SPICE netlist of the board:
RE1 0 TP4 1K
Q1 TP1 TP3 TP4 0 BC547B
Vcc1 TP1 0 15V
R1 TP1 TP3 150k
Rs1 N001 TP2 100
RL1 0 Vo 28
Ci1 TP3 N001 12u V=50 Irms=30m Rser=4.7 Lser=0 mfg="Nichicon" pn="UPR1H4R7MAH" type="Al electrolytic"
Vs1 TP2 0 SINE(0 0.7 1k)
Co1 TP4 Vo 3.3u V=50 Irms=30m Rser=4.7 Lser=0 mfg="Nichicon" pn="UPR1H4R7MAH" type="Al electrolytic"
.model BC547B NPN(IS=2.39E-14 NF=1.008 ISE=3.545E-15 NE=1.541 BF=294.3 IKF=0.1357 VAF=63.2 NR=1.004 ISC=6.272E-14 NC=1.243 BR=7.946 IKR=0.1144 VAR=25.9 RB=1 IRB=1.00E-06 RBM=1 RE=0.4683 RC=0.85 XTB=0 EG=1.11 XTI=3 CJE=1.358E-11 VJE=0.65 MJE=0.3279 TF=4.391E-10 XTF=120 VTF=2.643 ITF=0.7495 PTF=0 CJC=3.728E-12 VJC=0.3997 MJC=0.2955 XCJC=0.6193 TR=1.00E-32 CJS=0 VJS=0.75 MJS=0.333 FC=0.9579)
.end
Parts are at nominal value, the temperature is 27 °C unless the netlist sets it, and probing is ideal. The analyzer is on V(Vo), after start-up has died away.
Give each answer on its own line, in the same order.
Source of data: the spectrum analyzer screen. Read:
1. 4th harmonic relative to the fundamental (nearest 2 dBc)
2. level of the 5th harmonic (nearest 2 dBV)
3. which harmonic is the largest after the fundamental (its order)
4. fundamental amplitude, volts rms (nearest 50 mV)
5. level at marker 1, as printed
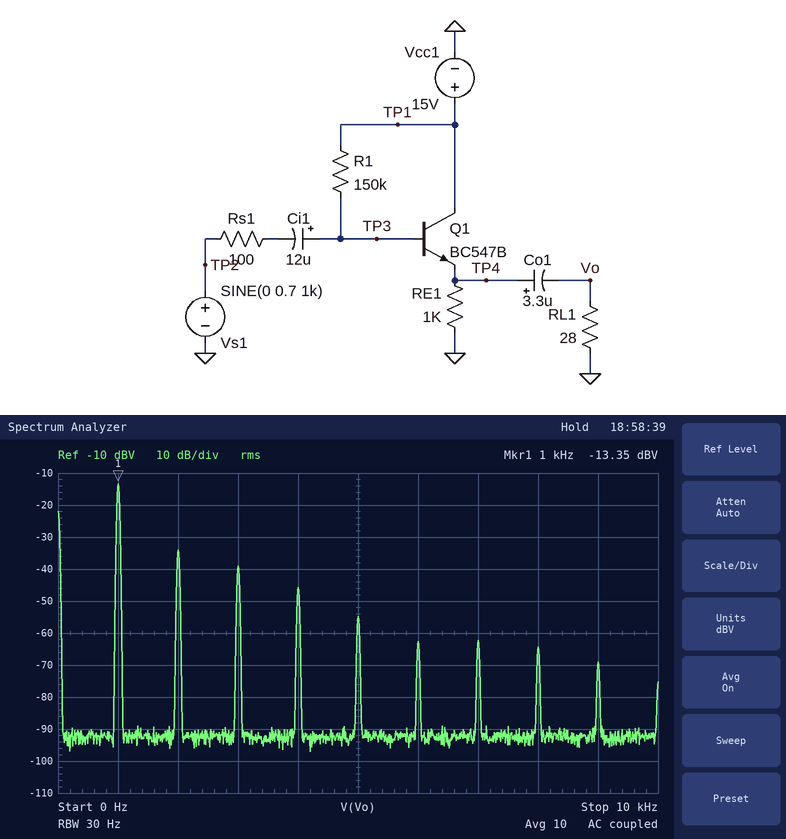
-32 dBc
-54 dBV
2
200 mV
-13.35 dBV
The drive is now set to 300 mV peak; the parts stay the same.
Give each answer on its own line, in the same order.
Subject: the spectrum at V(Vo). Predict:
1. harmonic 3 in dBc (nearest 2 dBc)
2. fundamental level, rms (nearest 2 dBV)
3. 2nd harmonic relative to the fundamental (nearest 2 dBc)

-54 dBc
-20 dBV
-40 dBc
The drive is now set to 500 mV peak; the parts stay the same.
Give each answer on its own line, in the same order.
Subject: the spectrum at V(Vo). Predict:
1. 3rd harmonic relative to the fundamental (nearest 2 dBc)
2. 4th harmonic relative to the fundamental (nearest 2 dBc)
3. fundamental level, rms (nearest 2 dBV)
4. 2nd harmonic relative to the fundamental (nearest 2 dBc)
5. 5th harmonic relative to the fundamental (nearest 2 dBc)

-40 dBc
-50 dBc
-16 dBV
-32 dBc
-58 dBc
